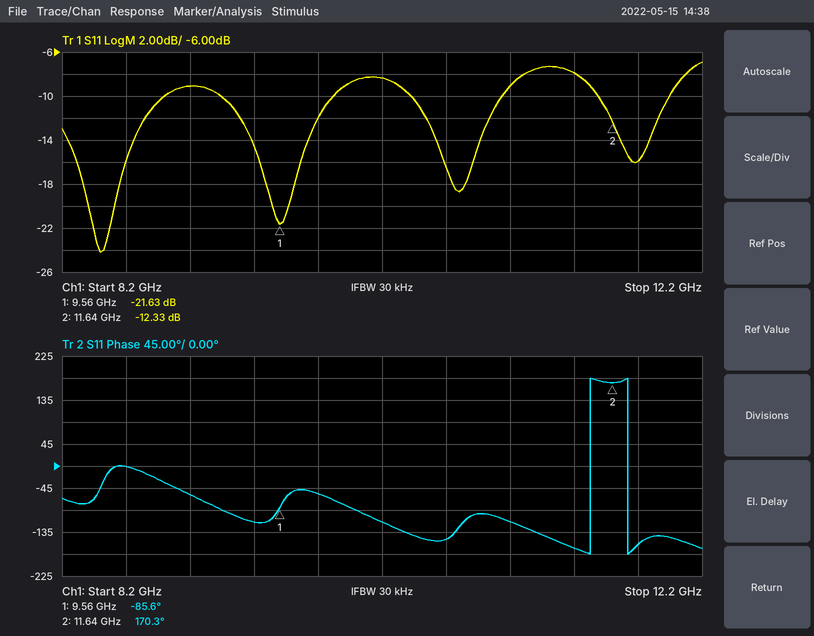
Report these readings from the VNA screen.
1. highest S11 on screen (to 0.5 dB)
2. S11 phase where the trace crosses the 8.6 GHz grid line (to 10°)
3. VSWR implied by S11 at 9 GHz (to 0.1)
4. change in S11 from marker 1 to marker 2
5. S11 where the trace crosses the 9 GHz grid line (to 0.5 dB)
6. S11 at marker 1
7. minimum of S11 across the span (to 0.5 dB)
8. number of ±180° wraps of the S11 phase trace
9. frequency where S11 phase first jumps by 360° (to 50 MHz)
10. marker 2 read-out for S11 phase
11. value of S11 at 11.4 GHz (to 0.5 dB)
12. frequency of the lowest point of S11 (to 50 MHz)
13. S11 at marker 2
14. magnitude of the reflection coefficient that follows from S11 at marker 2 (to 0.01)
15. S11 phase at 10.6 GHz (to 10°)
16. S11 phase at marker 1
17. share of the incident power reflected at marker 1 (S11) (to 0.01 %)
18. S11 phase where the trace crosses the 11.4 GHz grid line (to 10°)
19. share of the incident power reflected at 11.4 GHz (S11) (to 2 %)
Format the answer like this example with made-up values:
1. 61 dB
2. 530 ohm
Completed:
1. -7.0 dB
2. 0°
3. 2.1
4. 9.30 dB
5. -9.0 dB
6. -21.63 dB
7. -24.0 dB
8. 2
9. 11.50 GHz
10. 170.3°
11. -8.0 dB
12. 8.45 GHz
13. -12.33 dB
14. 0.24
15. -150°
16. -85.6°
17. 0.69 %
18. -170°
19. 16 %
